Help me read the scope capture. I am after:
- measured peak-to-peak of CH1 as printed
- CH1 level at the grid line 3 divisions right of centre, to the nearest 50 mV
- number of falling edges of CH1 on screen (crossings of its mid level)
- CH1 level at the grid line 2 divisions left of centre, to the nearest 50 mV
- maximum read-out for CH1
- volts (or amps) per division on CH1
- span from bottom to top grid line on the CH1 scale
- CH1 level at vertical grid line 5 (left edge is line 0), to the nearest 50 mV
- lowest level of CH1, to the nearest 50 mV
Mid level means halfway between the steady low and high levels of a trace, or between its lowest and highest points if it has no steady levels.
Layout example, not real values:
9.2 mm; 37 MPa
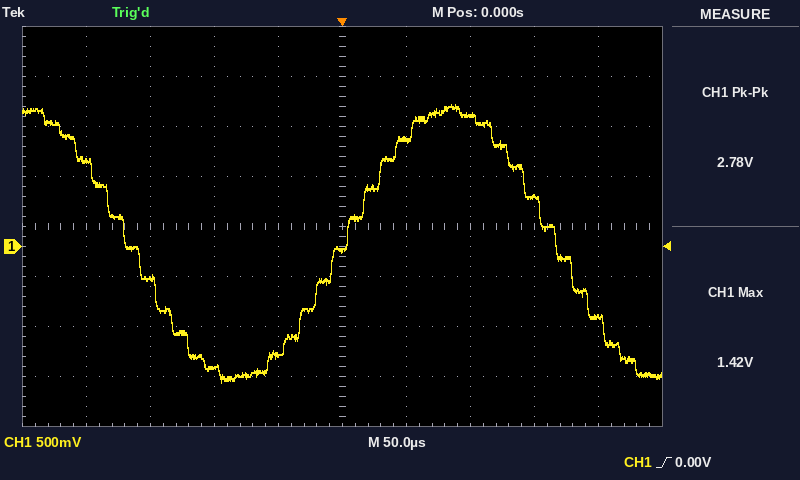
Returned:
2.78 V; 500 mV; 2; -1.20 V; 1.42 V; 500 mV; 4 V; -50 mV; -1.35 V
